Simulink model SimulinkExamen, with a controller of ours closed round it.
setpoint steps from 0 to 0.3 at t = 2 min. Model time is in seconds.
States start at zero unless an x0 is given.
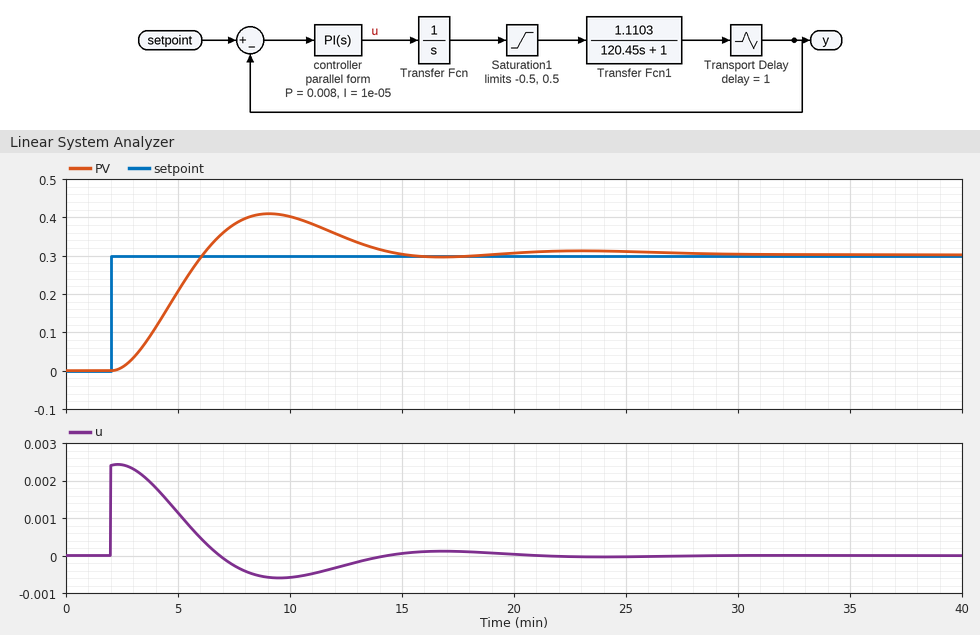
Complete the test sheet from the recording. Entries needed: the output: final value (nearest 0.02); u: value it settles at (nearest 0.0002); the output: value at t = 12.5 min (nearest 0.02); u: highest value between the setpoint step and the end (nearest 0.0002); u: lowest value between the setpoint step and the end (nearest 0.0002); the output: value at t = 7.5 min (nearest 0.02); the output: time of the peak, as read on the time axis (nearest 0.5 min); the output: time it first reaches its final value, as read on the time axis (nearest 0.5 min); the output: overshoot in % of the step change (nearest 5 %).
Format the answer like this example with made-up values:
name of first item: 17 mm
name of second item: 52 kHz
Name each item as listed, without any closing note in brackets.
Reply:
the output: final value: 0.30
u: value it settles at: 0.0000
the output: value at t = 12.5 min: 0.34
u: highest value between the setpoint step and the end: 0.0024
u: lowest value between the setpoint step and the end: -0.0006
the output: value at t = 7.5 min: 0.38
the output: time of the peak, as read on the time axis: 9.0 min
the output: time it first reaches its final value, as read on the time axis: 6.0 min
the output: overshoot in % of the step change: 35 %
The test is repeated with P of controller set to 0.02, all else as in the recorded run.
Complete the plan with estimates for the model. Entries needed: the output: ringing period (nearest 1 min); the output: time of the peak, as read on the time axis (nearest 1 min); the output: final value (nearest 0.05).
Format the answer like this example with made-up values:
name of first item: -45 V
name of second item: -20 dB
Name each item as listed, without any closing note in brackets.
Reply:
the output: ringing period: 8 min
the output: time of the peak, as read on the time axis: 6 min
the output: final value: 0.30
